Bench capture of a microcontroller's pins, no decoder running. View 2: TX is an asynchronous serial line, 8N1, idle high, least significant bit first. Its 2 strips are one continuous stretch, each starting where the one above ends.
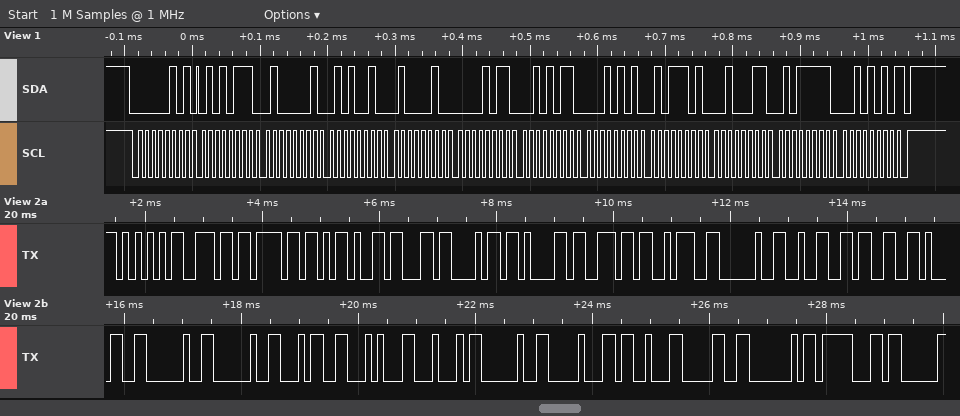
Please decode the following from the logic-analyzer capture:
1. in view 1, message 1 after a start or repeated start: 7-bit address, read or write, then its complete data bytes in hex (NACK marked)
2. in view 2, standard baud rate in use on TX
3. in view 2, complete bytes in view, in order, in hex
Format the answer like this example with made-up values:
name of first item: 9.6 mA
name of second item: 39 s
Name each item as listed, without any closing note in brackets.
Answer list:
in view 1, message 1 after a start or repeated start: 7-bit address, read or write, then its complete data bytes in hex: 0x02 read: 57 41 52 42 0B 2B 15 5D 23 5F 2A NACK
in view 2, standard baud rate in use on TX: 9600 baud
in view 2, complete bytes in view, in order, in hex: 55 6E 6F 2D 63 68 61 6E 3A 20 32 33 31 20 20 34 14 44 20 10 13 30 40 1F 03
